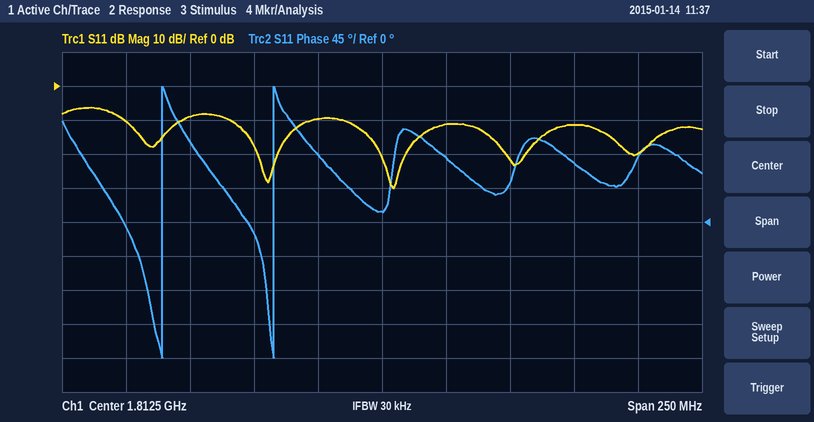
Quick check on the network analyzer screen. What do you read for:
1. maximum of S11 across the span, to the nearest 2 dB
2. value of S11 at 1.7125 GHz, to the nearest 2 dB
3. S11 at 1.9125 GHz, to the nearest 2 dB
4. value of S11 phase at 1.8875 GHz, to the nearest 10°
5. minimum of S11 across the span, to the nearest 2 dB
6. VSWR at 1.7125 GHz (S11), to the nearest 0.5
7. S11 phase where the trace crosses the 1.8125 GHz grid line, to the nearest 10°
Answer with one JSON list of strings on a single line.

["-6 dB", "-10 dB", "-20 dB", "80°", "-30 dB", "2.0", "10°"]
